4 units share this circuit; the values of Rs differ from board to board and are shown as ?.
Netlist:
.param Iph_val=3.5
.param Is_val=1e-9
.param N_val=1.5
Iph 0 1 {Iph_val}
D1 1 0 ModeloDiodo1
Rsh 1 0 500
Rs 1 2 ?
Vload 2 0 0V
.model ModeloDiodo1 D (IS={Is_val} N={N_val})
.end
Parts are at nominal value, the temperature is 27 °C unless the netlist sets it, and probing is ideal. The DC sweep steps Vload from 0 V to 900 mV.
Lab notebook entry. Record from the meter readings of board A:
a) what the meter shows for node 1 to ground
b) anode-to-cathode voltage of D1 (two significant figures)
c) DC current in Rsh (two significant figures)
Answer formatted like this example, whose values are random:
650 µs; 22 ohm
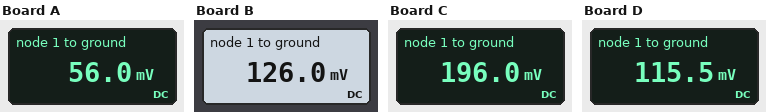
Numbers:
56.0 mV; 56 mV; 110 µA
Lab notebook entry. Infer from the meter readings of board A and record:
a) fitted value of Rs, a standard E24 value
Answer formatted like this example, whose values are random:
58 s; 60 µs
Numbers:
0.016 Ω
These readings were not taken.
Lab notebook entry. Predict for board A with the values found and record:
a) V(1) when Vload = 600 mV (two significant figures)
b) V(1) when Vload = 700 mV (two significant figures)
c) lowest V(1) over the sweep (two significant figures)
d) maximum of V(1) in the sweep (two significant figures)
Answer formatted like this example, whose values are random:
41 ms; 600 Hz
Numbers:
660 mV; 750 mV; 56 mV; 870 mV
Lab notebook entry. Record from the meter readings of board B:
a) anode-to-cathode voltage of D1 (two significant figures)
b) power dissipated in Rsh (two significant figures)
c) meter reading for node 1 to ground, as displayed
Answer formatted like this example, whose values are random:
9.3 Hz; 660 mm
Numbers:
130 mV; 32 µW; 126.0 mV
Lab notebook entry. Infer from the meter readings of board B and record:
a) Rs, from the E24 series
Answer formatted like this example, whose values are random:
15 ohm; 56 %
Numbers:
0.036 Ω
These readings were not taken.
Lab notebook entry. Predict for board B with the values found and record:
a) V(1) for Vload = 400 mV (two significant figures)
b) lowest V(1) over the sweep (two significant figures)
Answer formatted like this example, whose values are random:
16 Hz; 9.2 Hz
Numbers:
530 mV; 130 mV
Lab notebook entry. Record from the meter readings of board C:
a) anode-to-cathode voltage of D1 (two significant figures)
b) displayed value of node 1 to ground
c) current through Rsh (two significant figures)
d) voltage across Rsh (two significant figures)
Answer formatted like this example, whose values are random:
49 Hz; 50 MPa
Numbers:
200 mV; 196.0 mV; 390 µA; 200 mV
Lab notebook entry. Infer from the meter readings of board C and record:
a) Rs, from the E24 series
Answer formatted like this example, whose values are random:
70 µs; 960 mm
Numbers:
0.056 Ω
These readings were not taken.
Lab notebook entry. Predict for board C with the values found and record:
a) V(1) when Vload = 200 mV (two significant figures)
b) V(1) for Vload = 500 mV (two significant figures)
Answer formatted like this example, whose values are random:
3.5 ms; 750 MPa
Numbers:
400 mV; 690 mV
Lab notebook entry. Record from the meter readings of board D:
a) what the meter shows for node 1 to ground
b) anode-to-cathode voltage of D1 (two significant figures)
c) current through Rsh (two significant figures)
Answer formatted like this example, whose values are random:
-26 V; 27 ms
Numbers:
115.5 mV; 120 mV; 230 µA
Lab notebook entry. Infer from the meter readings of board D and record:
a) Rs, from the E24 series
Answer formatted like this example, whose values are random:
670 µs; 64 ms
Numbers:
0.033 Ω
